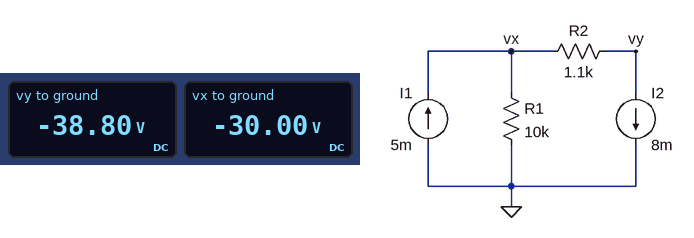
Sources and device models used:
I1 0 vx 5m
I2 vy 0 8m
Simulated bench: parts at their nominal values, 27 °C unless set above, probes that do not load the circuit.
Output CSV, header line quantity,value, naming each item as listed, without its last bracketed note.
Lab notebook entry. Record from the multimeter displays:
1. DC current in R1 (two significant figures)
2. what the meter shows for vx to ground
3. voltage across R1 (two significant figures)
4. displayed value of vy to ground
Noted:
quantity,value
DC current in R1,3.0 mA
what the meter shows for vx to ground,-30.00 V
voltage across R1,30 V
displayed value of vy to ground,-38.80 V
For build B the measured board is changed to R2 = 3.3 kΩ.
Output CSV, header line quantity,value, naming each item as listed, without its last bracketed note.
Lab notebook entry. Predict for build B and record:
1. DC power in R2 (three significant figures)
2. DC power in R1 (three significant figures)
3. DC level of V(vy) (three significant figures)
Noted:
quantity,value
DC power in R2,211 mW
DC power in R1,90.0 mW
DC level of V(vy),-56.4 V
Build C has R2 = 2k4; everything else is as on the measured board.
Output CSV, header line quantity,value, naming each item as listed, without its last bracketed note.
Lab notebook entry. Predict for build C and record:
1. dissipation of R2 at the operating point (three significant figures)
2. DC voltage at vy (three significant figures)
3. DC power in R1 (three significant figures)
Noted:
quantity,value
dissipation of R2 at the operating point,154 mW
DC voltage at vy,-49.2 V
DC power in R1,90.0 mW
